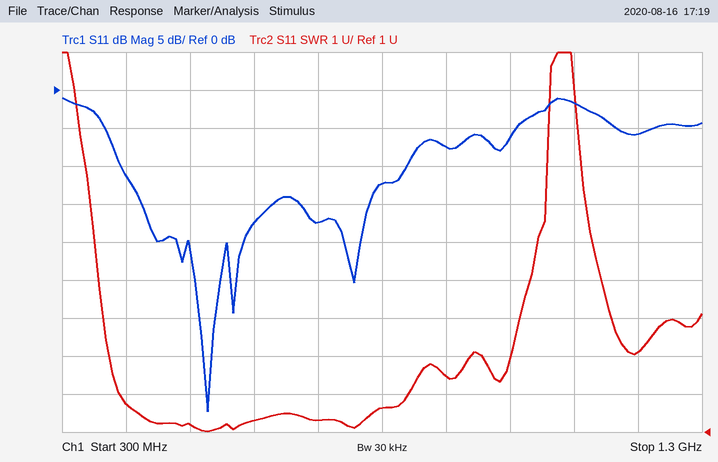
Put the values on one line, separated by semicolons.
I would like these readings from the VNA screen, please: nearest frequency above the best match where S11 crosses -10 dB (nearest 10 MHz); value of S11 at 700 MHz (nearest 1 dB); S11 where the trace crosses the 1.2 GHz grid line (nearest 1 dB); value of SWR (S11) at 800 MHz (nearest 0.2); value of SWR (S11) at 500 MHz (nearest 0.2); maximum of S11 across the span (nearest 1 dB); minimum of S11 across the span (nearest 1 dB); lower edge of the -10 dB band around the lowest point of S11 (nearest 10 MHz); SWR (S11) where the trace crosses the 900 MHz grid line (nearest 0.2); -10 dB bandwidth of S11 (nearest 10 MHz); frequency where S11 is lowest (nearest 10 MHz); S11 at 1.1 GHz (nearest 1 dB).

840 MHz; -17 dB; -6 dB; 1.6; 1.2; -1 dB; -42 dB; 390 MHz; 2.4; 450 MHz; 530 MHz; -2 dB
